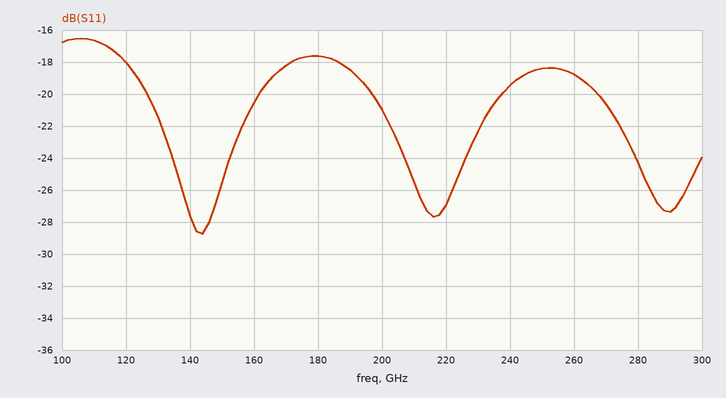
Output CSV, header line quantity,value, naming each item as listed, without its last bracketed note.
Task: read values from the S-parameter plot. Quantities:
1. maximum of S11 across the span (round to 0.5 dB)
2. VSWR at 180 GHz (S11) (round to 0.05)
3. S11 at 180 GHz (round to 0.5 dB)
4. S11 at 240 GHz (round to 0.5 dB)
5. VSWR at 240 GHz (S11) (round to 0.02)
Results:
quantity,value
maximum of S11 across the span,-16.5 dB
VSWR at 180 GHz (S11),1.30
S11 at 180 GHz,-17.5 dB
S11 at 240 GHz,-19.5 dB
VSWR at 240 GHz (S11),1.24
